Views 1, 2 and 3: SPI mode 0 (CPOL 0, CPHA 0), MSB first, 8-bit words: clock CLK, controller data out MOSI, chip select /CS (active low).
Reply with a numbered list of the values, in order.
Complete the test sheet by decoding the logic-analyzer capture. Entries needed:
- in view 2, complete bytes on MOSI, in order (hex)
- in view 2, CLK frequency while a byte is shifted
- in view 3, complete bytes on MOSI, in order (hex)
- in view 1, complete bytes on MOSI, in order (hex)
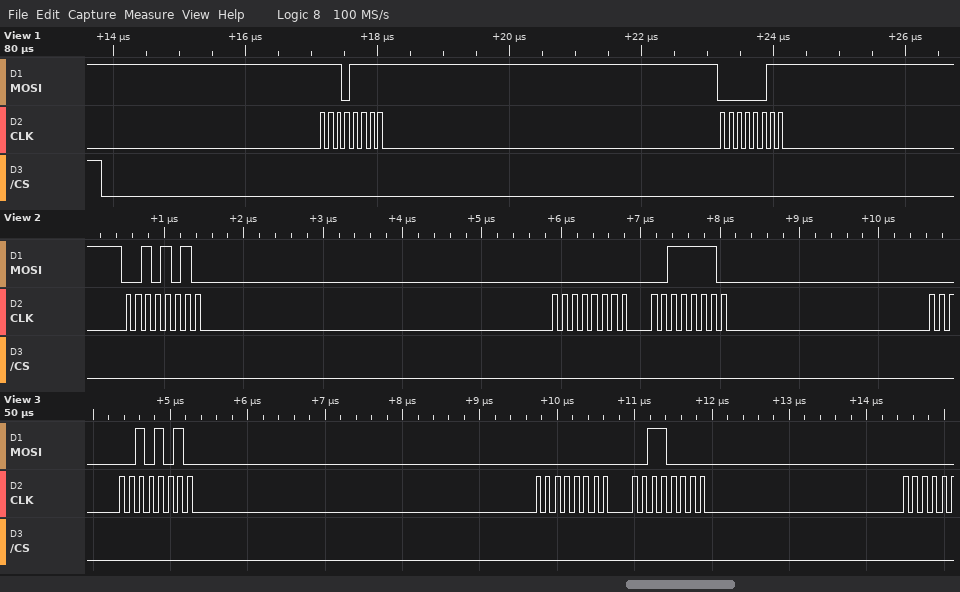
1. 2A 00 3E
2. 8 MHz
3. 2A 00 30
4. 0xEF 0x03
